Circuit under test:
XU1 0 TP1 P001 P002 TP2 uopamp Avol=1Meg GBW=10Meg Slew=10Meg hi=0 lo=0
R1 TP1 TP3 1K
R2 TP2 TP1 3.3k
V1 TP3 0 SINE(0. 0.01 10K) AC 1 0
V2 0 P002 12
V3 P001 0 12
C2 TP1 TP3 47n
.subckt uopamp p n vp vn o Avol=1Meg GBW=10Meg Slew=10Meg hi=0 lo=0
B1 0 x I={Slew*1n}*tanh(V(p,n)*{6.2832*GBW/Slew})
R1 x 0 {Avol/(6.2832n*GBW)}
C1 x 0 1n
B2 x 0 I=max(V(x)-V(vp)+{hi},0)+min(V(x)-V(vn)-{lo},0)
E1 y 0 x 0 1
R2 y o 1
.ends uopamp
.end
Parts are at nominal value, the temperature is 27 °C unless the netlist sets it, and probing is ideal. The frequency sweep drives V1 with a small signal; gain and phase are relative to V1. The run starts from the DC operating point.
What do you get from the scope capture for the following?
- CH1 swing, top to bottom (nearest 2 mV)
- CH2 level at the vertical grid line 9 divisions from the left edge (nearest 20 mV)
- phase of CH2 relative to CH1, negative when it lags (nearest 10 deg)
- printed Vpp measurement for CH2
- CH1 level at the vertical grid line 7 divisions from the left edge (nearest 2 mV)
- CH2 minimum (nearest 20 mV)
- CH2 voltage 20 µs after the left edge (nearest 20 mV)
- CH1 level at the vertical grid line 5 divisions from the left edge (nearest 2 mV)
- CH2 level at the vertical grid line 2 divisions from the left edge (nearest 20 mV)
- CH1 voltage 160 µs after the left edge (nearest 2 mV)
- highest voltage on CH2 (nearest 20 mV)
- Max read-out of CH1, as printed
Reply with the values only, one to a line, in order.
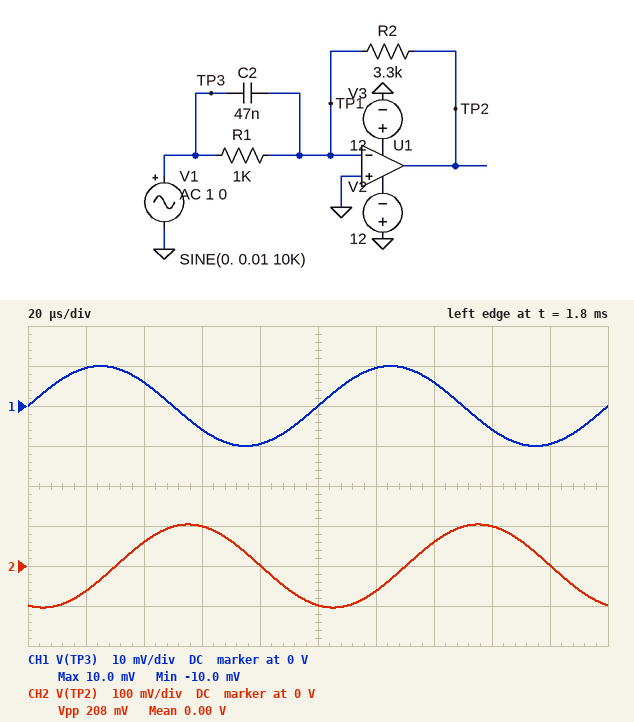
20 mV
0 V
-110 deg
208 mV
6 mV
-100 mV
-60 mV
0 V
60 mV
-6 mV
100 mV
10.0 mV
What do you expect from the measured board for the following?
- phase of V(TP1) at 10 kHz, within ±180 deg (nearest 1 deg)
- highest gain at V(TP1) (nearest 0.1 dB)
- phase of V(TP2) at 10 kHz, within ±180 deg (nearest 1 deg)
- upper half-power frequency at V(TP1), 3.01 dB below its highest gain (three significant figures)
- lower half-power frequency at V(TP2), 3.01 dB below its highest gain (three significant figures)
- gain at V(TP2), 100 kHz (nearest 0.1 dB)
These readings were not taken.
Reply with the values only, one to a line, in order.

161 deg
27.2 dB
-109 deg
104 kHz
99.1 kHz
65.8 dB
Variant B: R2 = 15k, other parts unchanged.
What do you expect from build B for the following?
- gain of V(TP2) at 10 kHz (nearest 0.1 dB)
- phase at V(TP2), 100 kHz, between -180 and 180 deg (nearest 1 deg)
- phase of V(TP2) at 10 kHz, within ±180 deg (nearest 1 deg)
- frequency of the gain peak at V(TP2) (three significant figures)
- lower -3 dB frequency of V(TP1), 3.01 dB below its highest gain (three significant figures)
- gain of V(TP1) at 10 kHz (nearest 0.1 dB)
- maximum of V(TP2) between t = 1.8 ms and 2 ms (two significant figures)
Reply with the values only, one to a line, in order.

33.8 dB
91 deg
-110 deg
47.5 kHz
45.9 kHz
-26.2 dB
490 mV
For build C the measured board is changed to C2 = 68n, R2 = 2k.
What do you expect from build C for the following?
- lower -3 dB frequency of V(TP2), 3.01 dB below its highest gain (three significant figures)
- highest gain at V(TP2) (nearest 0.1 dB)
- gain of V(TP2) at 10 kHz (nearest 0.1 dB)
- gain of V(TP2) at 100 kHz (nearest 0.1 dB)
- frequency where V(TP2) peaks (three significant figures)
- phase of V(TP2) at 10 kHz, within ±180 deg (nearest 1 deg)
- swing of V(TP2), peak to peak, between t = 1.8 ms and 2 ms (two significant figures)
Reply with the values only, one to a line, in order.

106 kHz
69.1 dB
18.9 dB
55.2 dB
108 kHz
-103 deg
180 mV
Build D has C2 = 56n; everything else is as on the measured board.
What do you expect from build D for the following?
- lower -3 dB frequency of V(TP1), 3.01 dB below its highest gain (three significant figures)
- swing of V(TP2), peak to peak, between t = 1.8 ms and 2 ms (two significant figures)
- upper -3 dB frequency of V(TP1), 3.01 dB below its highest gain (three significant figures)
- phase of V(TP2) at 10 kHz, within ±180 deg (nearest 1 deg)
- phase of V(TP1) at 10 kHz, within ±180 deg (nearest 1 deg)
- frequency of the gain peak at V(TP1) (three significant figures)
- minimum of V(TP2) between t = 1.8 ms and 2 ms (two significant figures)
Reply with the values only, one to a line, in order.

91.0 kHz
240 mV
94.7 kHz
-106 deg
164 deg
92.8 kHz
-120 mV
